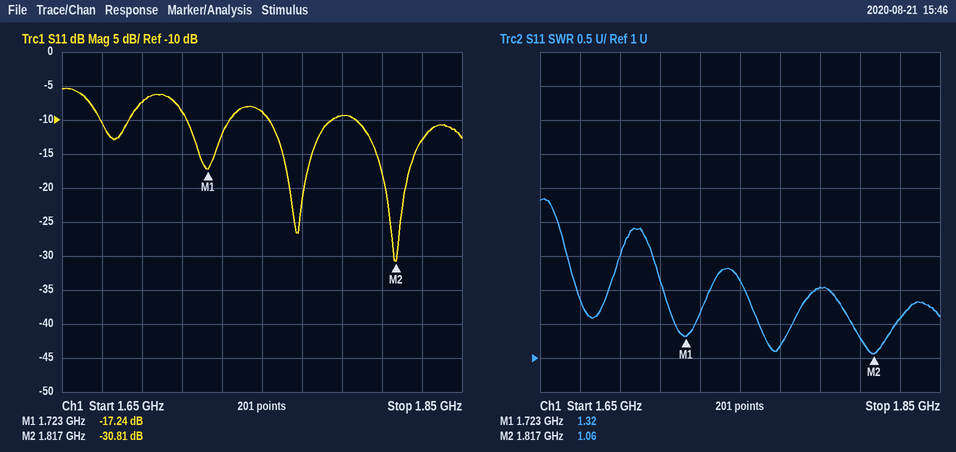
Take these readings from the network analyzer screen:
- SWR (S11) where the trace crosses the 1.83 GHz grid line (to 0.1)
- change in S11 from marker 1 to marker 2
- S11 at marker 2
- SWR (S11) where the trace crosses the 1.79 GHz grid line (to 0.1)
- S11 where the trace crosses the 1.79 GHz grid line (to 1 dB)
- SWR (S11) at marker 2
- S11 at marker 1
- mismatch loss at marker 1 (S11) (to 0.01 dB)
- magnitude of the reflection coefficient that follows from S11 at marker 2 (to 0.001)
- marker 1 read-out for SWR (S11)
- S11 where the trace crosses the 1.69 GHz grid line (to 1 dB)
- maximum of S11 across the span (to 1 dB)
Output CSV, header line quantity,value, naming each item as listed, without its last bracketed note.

quantity,value
SWR (S11) where the trace crosses the 1.83 GHz grid line,1.6
change in S11 from marker 1 to marker 2,-13.57 dB
S11 at marker 2,-30.81 dB
SWR (S11) where the trace crosses the 1.79 GHz grid line,2.0
S11 where the trace crosses the 1.79 GHz grid line,-9 dB
SWR (S11) at marker 2,1.06
S11 at marker 1,-17.24 dB
mismatch loss at marker 1 (S11),0.08 dB
magnitude of the reflection coefficient that follows from S11 at marker 2,0.029
marker 1 read-out for SWR,1.32
S11 where the trace crosses the 1.69 GHz grid line,-7 dB
maximum of S11 across the span,-5 dB
